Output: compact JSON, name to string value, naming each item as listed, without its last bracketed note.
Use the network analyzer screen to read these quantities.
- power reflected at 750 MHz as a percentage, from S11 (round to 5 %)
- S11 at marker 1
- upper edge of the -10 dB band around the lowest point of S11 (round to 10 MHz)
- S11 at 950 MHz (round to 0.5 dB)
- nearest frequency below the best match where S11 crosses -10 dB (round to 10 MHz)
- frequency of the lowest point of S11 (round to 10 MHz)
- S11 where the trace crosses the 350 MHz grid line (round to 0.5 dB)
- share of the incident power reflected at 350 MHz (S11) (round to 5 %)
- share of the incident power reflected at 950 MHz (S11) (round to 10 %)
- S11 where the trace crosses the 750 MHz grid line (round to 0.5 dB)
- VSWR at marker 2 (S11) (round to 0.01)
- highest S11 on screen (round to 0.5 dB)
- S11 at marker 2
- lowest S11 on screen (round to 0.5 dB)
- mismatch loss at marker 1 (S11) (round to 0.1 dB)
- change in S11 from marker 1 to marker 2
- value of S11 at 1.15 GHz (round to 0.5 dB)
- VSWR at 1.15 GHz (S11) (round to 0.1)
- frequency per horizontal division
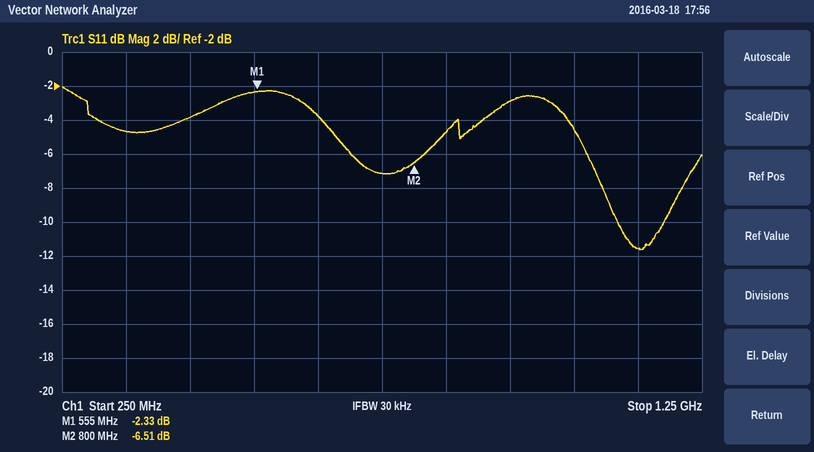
{"power reflected at 750 MHz as a percentage, from S11": "20 %", "S11 at marker 1": "-2.33 dB", "upper edge of the -10 dB band around the lowest point of S11": "1.19 GHz", "S11 at 950 MHz": "-3.0 dB", "nearest frequency below the best match where S11 crosses -10 dB": "1.12 GHz", "frequency of the lowest point of S11": "1.15 GHz", "S11 where the trace crosses the 350 MHz grid line": "-4.5 dB", "share of the incident power reflected at 350 MHz (S11)": "35 %", "share of the incident power reflected at 950 MHz (S11)": "50 %", "S11 where the trace crosses the 750 MHz grid line": "-7.0 dB", "VSWR at marker 2 (S11)": "2.79", "highest S11 on screen": "-2.0 dB", "S11 at marker 2": "-6.51 dB", "lowest S11 on screen": "-11.5 dB", "mismatch loss at marker 1 (S11)": "3.8 dB", "change in S11 from marker 1 to marker 2": "-4.18 dB", "value of S11 at 1.15 GHz": "-11.5 dB", "VSWR at 1.15 GHz (S11)": "1.7", "frequency per horizontal division": "100 MHz"}
